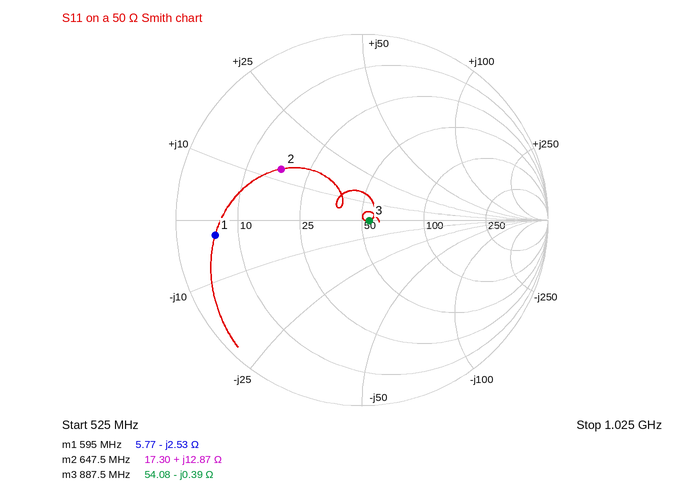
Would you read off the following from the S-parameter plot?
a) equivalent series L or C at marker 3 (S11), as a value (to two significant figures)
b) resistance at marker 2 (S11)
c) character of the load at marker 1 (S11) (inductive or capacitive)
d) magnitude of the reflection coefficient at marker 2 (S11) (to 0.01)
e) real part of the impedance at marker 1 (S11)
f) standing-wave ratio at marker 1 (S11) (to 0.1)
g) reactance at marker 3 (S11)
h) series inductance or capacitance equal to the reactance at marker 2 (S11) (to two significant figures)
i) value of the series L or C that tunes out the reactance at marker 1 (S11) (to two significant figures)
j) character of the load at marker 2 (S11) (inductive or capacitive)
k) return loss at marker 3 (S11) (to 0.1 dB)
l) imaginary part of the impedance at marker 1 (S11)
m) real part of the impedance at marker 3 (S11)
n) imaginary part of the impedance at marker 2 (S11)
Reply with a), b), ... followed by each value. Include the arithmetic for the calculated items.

a) C = 1/(2π × 887.5 MHz × 0.39 Ω) ≈ 460 pF
b) 17.30 Ω
c) capacitive
d) 0.51
e) 5.77 Ω
f) 8.7
g) -0.39 Ω
h) L = 12.87 Ω/(2π × 647.5 MHz) ≈ 3.2 nH
i) L = 2.53 Ω/(2π × 595 MHz) ≈ 677 pH, so 680 pH to two significant figures
j) inductive
k) 28.1 dB
l) -2.53 Ω
m) 54.08 Ω
n) +12.87 Ω
